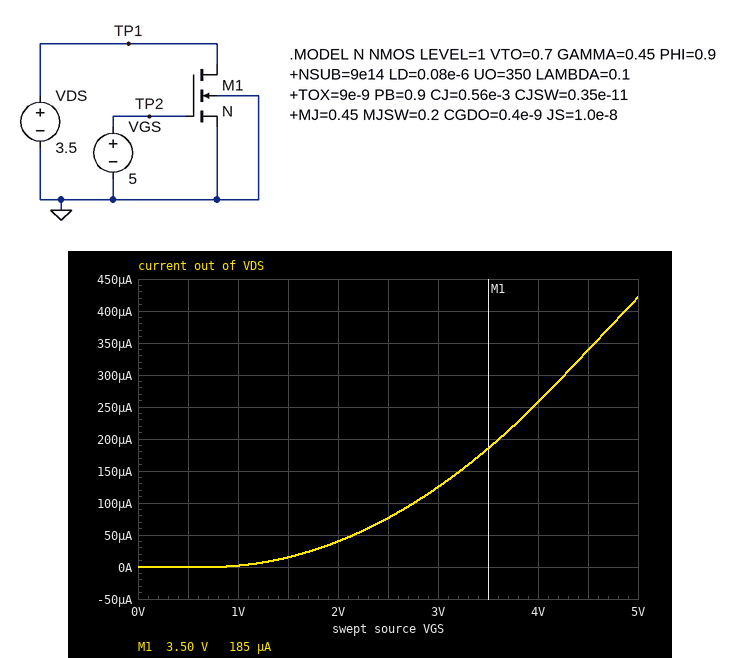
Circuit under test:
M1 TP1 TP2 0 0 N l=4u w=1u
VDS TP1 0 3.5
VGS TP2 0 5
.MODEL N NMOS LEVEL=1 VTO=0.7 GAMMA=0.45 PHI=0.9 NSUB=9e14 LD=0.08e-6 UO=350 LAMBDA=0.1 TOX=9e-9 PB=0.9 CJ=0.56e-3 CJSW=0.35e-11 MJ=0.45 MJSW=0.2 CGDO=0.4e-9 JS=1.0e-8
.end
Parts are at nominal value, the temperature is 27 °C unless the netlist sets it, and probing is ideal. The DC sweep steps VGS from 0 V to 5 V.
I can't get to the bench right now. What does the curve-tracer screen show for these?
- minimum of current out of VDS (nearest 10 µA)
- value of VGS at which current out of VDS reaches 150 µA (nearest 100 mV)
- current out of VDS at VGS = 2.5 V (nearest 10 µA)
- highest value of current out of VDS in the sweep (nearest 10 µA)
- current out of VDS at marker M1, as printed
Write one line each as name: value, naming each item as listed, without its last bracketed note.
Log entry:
minimum of current out of VDS: 0 A
value of VGS at which current out of VDS reaches 150 µA: 3.2 V
current out of VDS at VGS = 2.5 V: 80 µA
highest value of current out of VDS in the sweep: 420 µA
current out of VDS at marker M1, as printed: 185 µA
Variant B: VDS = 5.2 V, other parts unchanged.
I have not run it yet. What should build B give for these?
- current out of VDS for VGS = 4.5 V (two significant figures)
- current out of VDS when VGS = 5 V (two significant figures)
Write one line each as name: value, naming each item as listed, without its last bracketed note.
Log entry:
current out of VDS for VGS = 4.5 V: 380 µA
current out of VDS when VGS = 5 V: 490 µA
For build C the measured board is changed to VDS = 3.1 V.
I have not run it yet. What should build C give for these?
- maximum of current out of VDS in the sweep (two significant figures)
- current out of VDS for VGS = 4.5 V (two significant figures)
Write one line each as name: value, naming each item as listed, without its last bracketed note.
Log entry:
maximum of current out of VDS in the sweep: 390 µA
current out of VDS for VGS = 4.5 V: 320 µA
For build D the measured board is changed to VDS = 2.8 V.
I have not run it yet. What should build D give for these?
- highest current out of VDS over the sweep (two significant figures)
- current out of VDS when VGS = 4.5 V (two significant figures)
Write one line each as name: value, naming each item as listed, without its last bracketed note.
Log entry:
highest current out of VDS over the sweep: 360 µA
current out of VDS when VGS = 4.5 V: 300 µA
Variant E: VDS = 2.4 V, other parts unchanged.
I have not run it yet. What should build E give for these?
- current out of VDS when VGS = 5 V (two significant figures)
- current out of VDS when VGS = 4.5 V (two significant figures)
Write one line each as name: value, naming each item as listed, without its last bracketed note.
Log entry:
current out of VDS when VGS = 5 V: 320 µA
current out of VDS when VGS = 4.5 V: 270 µA
